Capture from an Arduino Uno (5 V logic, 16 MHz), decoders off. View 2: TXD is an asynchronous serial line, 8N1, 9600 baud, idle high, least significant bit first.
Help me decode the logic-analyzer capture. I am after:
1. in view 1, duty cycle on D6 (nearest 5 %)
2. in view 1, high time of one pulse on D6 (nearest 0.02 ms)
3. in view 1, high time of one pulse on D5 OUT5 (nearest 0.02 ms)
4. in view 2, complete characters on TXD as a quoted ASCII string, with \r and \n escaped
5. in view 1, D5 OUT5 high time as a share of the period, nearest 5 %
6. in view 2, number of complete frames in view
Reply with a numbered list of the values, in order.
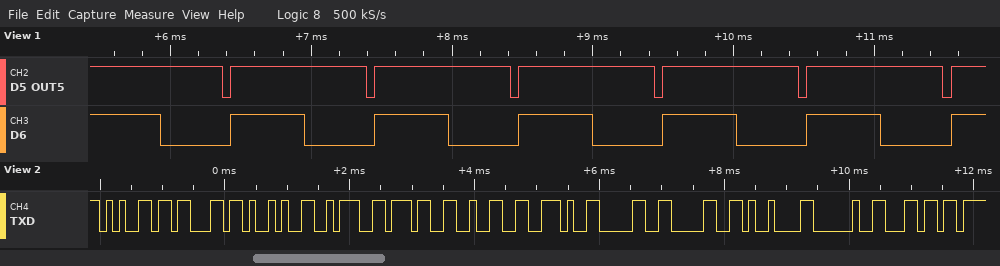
1. 50 %
2. 0.52 ms
3. 0.96 ms
4. "ec):72.00\t l"
5. 95 %
6. 12
